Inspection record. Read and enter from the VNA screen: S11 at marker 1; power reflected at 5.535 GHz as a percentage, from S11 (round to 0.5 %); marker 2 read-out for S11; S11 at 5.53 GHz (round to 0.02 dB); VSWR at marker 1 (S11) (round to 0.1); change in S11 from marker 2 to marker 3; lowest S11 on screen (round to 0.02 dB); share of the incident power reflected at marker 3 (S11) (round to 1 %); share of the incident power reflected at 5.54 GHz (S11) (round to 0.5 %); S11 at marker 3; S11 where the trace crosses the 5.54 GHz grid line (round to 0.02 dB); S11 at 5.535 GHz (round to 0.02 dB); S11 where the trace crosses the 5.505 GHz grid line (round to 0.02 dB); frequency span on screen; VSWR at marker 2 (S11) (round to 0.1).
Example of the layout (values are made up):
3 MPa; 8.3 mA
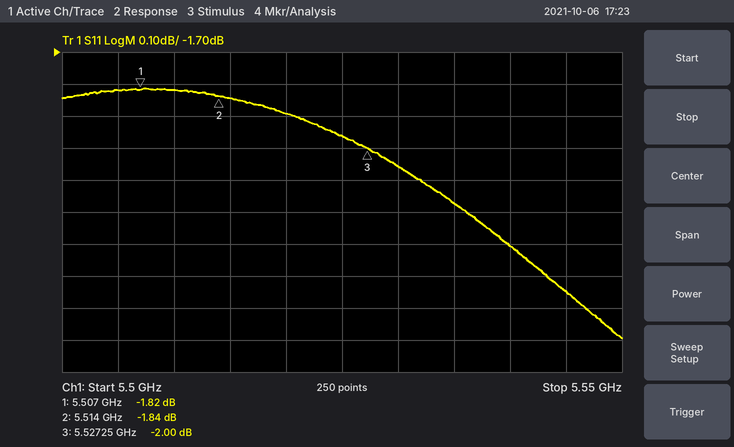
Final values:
-1.82 dB; 60.5 %; -1.84 dB; -2.06 dB; 9.6; -0.16 dB; -2.60 dB; 63 %; 59.0 %; -2.00 dB; -2.30 dB; -2.18 dB; -1.82 dB; 50 MHz; 9.5
